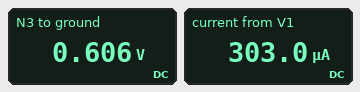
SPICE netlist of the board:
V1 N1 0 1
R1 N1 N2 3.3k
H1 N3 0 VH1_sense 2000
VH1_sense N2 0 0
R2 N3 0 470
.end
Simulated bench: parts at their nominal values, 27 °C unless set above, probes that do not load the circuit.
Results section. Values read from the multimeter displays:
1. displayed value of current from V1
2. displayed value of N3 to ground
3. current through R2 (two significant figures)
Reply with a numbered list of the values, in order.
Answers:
1. 303.0 µA
2. 0.606 V
3. 1.3 mA
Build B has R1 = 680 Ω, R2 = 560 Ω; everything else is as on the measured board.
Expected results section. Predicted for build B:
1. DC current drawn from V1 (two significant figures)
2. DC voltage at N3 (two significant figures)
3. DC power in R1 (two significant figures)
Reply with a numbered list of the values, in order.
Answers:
1. 1.5 mA
2. 2.9 V
3. 1.5 mW
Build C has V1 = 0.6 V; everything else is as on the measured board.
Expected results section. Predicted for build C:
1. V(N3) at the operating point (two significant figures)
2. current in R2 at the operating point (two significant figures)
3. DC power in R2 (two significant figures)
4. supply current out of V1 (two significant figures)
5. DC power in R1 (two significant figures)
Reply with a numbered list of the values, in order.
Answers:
1. 360 mV
2. 770 µA
3. 280 µW
4. 180 µA
5. 110 µW
